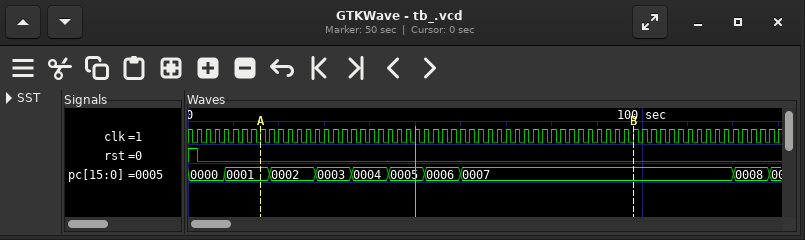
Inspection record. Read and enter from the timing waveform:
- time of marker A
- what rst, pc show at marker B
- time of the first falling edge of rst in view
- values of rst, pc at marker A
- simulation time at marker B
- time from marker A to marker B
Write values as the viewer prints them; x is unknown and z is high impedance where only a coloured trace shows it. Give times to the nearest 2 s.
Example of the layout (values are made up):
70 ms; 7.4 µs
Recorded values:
16 s; rst=0, pc=0007; 2 s; rst=0, pc=0001; 98 s; 82 s
